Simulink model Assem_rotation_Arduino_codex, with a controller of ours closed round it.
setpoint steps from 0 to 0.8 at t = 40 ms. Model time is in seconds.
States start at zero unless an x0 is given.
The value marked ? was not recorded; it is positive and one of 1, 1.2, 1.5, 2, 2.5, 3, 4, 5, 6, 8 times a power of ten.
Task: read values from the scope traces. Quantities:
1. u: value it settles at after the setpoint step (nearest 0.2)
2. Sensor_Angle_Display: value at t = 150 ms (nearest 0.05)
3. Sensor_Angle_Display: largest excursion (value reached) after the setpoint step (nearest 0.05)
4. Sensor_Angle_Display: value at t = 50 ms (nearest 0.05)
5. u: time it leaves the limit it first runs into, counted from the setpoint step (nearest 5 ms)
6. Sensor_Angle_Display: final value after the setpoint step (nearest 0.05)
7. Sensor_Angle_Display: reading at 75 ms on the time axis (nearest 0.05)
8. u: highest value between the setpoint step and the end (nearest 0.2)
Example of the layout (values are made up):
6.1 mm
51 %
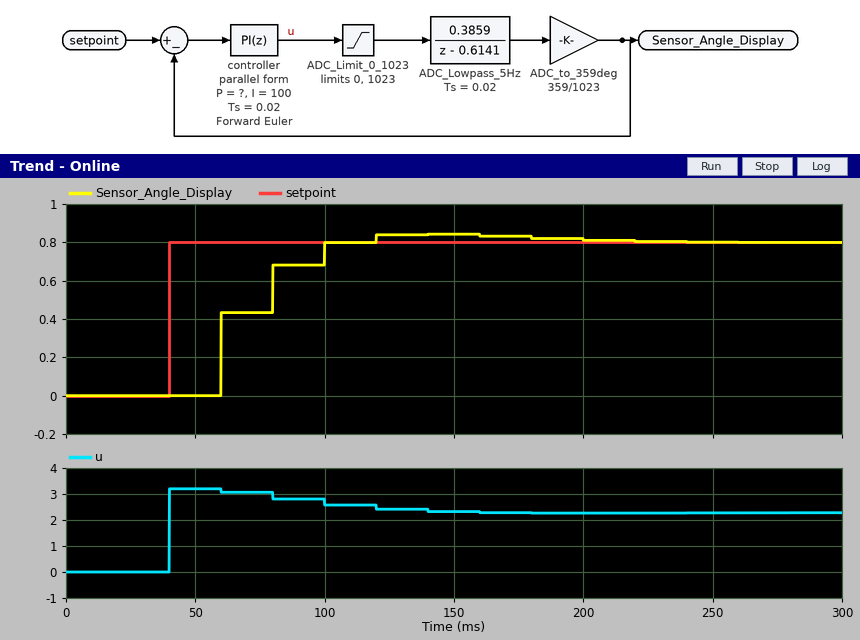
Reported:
2.2
0.85
0.85
0.00
20 ms
0.80
0.45
3.2
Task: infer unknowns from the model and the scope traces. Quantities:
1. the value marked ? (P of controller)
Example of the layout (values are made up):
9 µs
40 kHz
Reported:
4
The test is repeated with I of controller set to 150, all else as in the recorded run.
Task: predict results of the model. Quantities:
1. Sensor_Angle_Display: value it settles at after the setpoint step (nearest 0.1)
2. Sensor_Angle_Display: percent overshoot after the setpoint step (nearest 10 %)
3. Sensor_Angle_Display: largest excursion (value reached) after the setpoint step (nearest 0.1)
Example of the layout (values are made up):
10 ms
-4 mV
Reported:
0.8
20 %
1.0
